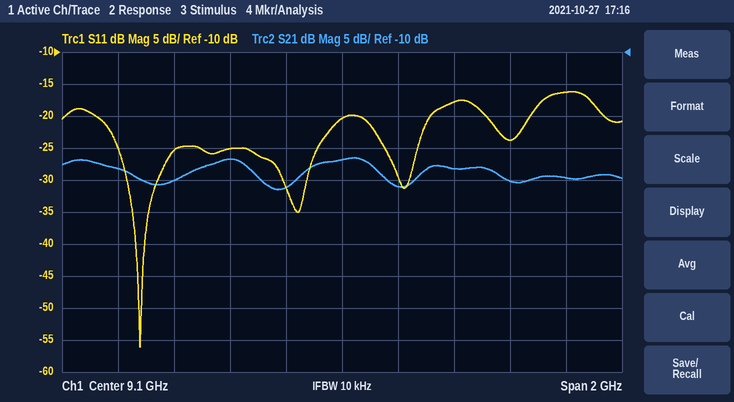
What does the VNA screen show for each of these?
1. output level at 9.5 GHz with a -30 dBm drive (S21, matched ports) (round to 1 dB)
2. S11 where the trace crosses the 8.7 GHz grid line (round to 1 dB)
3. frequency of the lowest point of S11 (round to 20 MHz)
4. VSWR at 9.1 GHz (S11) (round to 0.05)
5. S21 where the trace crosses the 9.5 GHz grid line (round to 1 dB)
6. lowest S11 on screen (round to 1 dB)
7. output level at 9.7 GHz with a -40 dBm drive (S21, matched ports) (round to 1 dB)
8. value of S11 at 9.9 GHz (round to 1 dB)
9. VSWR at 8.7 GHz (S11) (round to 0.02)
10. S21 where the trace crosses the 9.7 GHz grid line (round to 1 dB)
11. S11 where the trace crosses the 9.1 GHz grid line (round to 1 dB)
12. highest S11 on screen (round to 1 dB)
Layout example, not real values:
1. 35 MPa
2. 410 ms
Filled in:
1. -58 dBm
2. -25 dB
3. 8.38 GHz
4. 1.20
5. -28 dB
6. -56 dB
7. -70 dBm
8. -16 dB
9. 1.12
10. -30 dB
11. -20 dB
12. -16 dB
